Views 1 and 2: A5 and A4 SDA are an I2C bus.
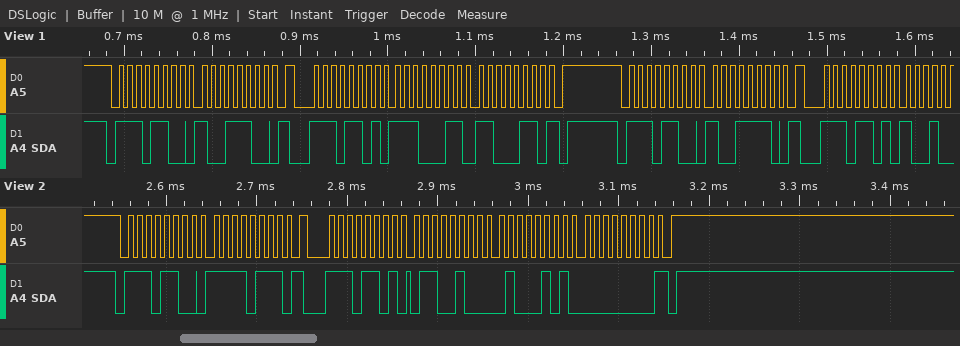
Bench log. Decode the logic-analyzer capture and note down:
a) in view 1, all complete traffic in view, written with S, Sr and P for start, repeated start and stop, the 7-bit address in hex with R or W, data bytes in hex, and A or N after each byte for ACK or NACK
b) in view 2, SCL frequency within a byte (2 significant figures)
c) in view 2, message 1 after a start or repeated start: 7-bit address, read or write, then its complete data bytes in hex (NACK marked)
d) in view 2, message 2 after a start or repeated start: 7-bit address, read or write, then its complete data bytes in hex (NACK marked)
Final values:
S 76W A 9C A Sr 76R A E3 A C6 N P S 76W A 9E A Sr 76R A
100 kHz
0x76 write: F7
0x76 read: 64 45 00 NACK
